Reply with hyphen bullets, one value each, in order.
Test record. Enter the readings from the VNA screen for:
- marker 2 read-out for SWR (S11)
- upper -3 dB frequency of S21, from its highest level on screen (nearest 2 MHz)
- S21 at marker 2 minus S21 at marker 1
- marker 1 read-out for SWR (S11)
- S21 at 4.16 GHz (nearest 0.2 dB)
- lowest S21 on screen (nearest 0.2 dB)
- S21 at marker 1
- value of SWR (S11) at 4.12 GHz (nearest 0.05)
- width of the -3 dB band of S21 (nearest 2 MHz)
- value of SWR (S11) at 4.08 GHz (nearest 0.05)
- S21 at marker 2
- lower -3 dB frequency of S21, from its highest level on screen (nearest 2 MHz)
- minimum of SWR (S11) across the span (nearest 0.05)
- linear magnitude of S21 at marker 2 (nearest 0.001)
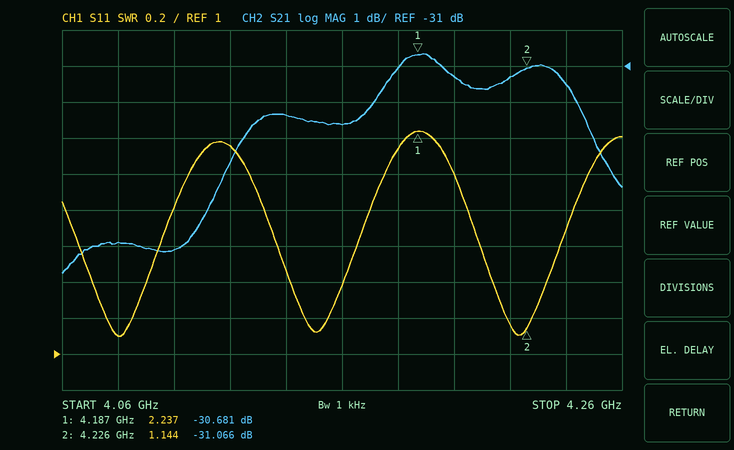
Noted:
- 1.144
- 4.254 GHz
- -0.385 dB
- 2.237
- -32.6 dB
- -36.8 dB
- -30.681 dB
- 2.15
- 134 MHz
- 1.10
- -31.066 dB
- 4.120 GHz
- 1.10
- 0.028
